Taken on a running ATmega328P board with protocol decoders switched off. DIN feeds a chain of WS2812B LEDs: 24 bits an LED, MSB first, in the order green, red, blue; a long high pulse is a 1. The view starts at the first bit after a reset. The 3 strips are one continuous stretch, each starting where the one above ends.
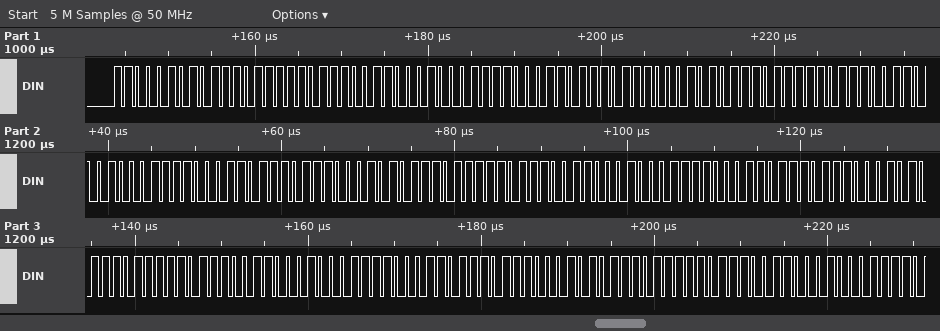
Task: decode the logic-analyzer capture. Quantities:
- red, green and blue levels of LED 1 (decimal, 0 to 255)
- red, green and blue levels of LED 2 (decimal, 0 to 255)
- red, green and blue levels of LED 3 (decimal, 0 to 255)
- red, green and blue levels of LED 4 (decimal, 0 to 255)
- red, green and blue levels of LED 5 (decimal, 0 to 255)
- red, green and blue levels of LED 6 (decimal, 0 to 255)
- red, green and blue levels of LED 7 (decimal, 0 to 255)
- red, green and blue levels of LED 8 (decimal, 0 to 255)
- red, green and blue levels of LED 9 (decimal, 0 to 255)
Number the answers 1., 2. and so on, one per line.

1. 119, 197, 220
2. 120, 196, 221
3. 119, 197, 220
4. 120, 196, 221
5. 119, 197, 220
6. 120, 196, 221
7. 119, 197, 220
8. 120, 196, 221
9. 119, 197, 220
